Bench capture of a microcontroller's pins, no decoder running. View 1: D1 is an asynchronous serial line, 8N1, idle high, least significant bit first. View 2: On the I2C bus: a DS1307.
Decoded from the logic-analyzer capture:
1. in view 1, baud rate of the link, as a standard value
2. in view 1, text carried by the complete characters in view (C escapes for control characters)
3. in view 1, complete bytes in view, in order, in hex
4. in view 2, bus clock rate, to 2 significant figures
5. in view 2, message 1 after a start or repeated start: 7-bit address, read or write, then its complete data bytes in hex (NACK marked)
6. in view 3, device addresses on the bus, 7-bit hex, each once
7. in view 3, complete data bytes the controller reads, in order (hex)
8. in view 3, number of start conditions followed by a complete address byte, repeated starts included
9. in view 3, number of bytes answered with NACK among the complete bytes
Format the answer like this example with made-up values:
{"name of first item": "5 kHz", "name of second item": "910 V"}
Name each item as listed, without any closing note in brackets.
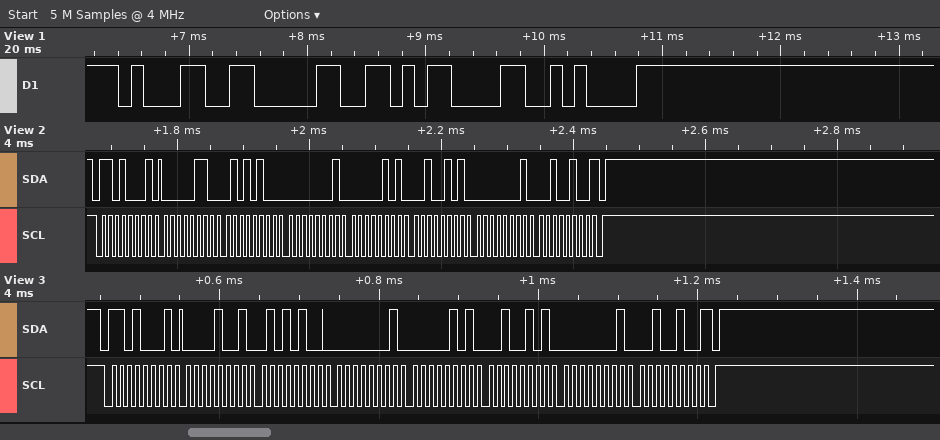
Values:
{"in view 1, baud rate of the link, as a standard value": "9600 baud", "in view 1, text carried by the complete characters in view": "\"10\\r\\n\"", "in view 1, complete bytes in view, in order, in hex": "31 30 0D 0A", "in view 2, bus clock rate, to 2 significant figures": "100 kHz", "in view 2, message 1 after a start or repeated start: 7-bit address, read or write, then its complete data bytes in hex": "0x68 read: 06 54 01 05 25 01 24 NACK", "in view 3, device addresses on the bus, 7-bit hex, each once": "0x68", "in view 3, complete data bytes the controller reads, in order": "09 54 01 05 25 01 24", "in view 3, number of start conditions followed by a complete address byte, repeated starts included": "1", "in view 3, number of bytes answered with NACK among the complete bytes": "1"}
